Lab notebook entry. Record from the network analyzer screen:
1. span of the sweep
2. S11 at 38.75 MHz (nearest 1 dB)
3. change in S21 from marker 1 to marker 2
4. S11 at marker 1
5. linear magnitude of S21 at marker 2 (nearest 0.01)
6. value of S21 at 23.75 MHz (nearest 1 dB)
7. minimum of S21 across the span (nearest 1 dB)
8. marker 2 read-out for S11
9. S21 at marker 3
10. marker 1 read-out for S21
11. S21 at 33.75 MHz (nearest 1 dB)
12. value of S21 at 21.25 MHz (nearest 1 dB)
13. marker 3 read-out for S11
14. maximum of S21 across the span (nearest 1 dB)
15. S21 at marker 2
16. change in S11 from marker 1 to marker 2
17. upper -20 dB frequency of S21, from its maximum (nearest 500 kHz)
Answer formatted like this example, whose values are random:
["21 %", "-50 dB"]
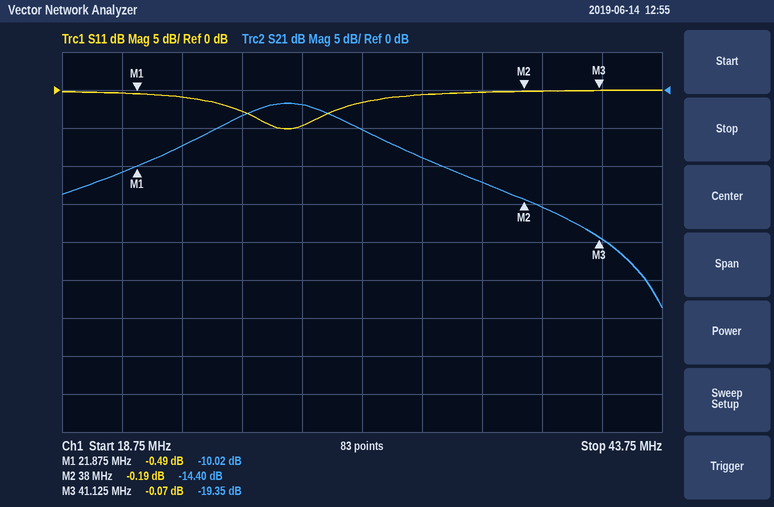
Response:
["25 MHz", "0 dB", "-4.38 dB", "-0.49 dB", "0.19", "-7 dB", "-29 dB", "-0.19 dB", "-19.35 dB", "-10.02 dB", "-9 dB", "-11 dB", "-0.07 dB", "-2 dB", "-14.40 dB", "0.30 dB", "42.0 MHz"]
